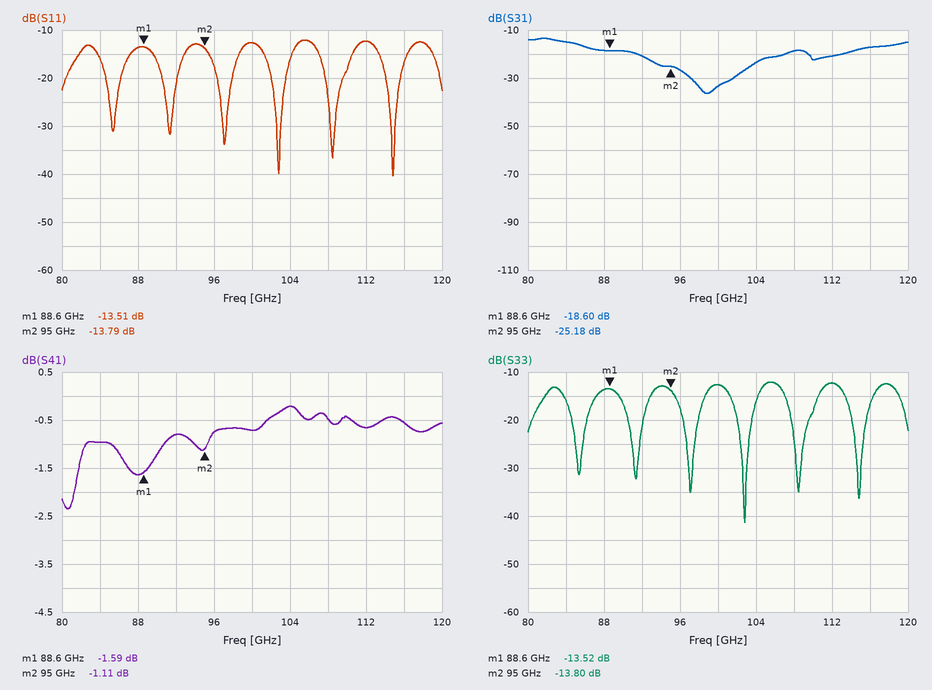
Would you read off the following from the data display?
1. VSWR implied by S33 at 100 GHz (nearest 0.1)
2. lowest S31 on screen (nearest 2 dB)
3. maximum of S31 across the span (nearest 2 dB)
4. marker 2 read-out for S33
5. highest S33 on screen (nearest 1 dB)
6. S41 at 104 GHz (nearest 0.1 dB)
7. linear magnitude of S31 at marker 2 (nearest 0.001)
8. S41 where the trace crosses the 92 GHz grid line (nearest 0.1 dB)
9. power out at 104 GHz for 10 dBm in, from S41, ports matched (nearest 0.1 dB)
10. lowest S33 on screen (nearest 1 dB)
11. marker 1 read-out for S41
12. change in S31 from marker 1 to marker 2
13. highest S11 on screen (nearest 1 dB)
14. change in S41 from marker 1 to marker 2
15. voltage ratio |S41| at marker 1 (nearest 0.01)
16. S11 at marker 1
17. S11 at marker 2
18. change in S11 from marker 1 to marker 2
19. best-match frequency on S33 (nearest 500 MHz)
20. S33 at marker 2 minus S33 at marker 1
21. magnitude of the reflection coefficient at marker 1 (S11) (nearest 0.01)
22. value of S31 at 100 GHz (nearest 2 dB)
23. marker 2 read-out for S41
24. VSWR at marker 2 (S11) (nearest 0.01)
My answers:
1.6
-36 dB
-14 dB
-13.80 dB
-12 dB
-0.2 dB
0.055
-0.8 dB
9.8 dBm
-41 dB
-1.59 dB
-6.58 dB
-12 dB
0.48 dB
0.83
-13.51 dB
-13.79 dB
-0.28 dB
103.0 GHz
-0.28 dB
0.21
-34 dB
-1.11 dB
1.51
